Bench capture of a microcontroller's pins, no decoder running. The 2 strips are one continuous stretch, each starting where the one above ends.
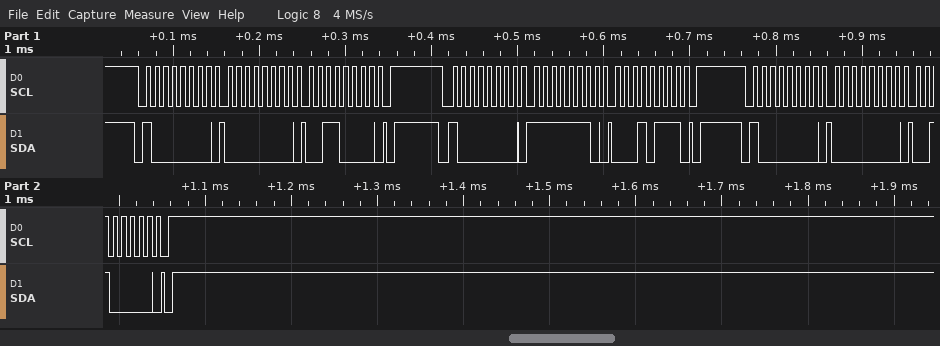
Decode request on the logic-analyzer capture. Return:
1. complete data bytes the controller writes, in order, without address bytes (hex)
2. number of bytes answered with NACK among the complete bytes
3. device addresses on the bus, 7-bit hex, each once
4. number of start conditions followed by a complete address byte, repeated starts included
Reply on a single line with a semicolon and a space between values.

00 30 FE 17 00 20; 0; 0x40; 3
